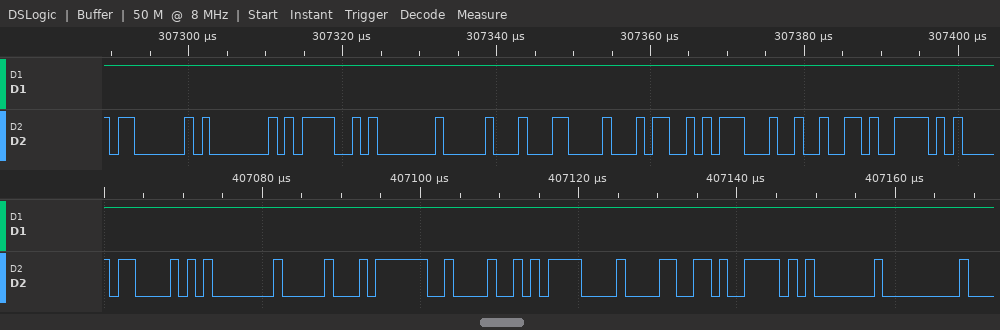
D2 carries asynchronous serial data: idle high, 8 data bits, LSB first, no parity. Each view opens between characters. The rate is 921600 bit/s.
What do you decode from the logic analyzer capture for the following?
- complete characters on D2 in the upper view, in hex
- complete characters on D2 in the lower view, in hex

03, 01, 3D, 01, 10, 0C, 34, 1D, 92, 79
43, 01, 10, 3F, 48, 0F, 98, 79, 01, 00
